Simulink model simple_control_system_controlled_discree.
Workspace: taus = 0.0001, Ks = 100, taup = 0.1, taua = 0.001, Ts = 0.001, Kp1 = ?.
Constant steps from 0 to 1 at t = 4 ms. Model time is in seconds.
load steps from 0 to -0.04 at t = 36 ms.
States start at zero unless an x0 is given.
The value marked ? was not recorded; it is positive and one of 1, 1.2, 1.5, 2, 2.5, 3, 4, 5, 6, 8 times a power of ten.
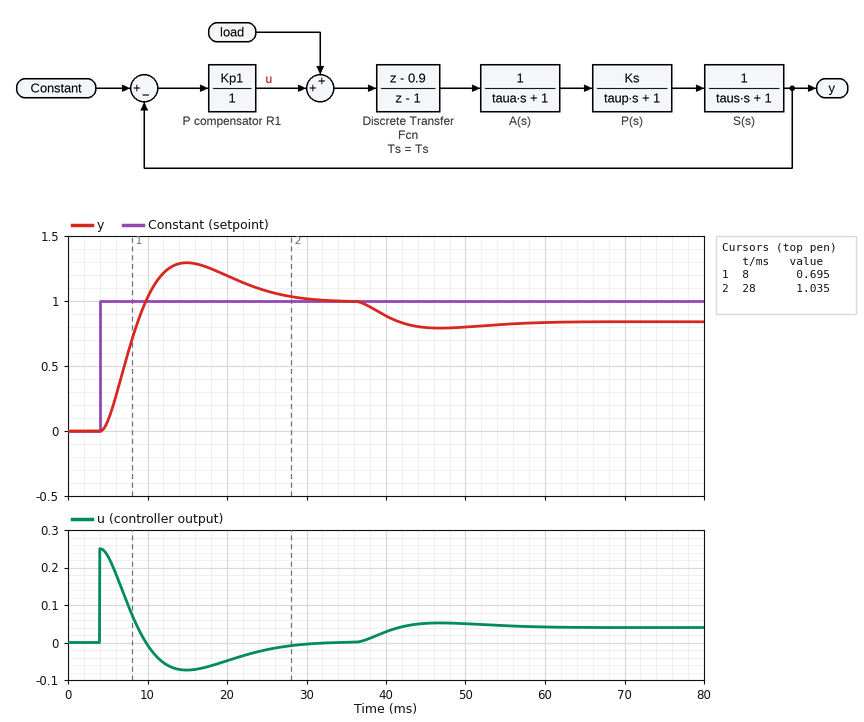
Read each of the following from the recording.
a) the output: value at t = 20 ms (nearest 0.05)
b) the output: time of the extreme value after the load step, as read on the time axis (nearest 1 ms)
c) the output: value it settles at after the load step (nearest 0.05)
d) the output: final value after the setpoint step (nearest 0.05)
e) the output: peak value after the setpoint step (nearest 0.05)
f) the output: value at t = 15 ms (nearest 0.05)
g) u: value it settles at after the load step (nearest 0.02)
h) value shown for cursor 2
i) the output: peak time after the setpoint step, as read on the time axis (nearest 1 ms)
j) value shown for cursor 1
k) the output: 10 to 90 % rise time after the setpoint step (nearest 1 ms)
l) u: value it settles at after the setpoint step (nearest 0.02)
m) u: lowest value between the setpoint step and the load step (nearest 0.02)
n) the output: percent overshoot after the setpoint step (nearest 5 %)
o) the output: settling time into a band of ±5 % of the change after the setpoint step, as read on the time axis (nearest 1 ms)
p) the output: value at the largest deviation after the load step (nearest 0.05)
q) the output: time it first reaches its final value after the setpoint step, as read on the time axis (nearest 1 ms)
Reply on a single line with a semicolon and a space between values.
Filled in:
1.20; 47 ms; 0.85; 1.00; 1.30; 1.30; 0.04; 1.035; 15 ms; 0.695; 4 ms; 0.00; -0.08; 30 %; 27 ms; 0.80; 10 ms
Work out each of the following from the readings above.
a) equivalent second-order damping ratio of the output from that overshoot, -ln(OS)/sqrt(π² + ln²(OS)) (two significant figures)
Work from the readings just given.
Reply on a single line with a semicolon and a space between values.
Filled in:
0.36
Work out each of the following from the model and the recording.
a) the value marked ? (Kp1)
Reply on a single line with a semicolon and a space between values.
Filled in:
0.25
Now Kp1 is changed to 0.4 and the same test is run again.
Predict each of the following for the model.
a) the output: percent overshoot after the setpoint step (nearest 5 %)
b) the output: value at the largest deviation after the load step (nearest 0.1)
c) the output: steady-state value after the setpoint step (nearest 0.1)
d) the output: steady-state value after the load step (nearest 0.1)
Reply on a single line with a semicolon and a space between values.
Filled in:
35 %; 0.9; 1.0; 0.9
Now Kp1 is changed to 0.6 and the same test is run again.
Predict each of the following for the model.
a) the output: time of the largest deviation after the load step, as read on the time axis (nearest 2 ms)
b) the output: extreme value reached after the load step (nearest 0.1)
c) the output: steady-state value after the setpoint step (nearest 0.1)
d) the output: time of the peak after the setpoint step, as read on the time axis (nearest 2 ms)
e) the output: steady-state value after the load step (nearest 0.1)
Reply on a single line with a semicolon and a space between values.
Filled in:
42 ms; 0.9; 1.0; 10 ms; 0.9
